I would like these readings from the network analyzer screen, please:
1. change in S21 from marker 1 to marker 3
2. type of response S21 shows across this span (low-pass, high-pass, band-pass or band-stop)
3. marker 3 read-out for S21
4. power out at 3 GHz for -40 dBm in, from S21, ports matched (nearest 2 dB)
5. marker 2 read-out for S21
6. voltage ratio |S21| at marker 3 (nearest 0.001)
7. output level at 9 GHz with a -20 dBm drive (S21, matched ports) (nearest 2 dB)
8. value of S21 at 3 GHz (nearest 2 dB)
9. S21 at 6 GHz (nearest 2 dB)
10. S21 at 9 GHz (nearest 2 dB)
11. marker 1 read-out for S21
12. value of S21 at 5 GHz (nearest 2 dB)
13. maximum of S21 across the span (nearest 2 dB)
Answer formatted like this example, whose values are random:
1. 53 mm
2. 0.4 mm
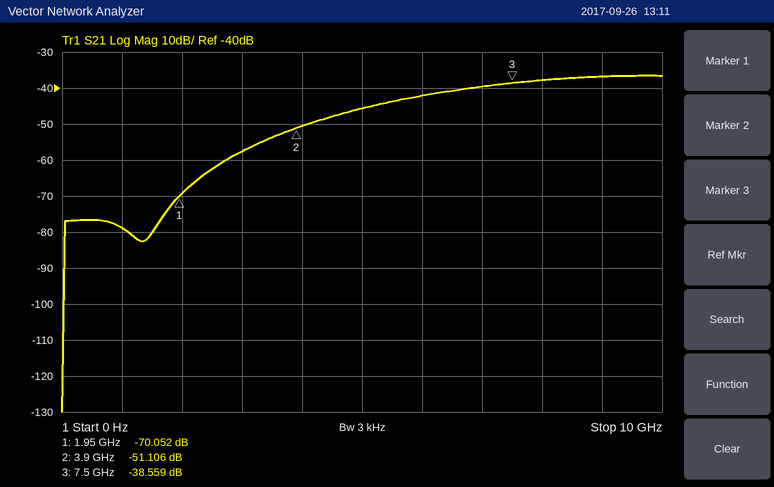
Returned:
1. 31.493 dB
2. high-pass
3. -38.559 dB
4. -98 dBm
5. -51.106 dB
6. 0.012
7. -56 dBm
8. -58 dB
9. -42 dB
10. -36 dB
11. -70.052 dB
12. -46 dB
13. -36 dB
